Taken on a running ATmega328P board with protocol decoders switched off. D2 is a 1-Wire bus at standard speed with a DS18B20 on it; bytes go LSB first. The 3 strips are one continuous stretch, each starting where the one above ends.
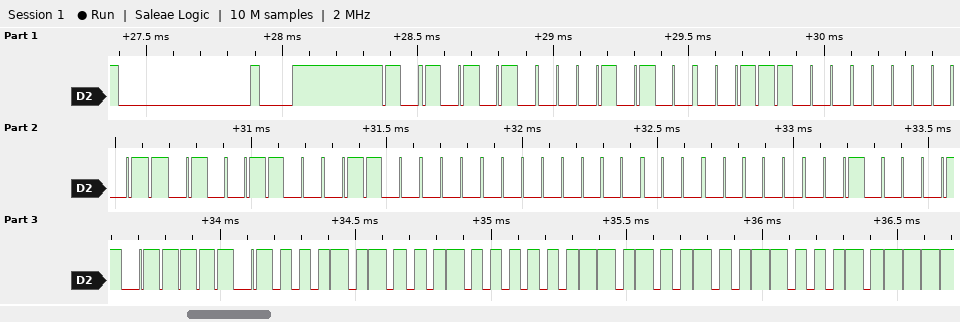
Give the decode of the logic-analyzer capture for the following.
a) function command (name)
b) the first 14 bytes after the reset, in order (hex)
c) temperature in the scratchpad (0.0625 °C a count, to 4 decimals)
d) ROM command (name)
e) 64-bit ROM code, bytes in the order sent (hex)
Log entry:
Read Scratchpad
55 28 1C C0 32 06 00 00 84 BE 28 02 4B 46
34.5000 °C
Match ROM
28 1C C0 32 06 00 00 84
